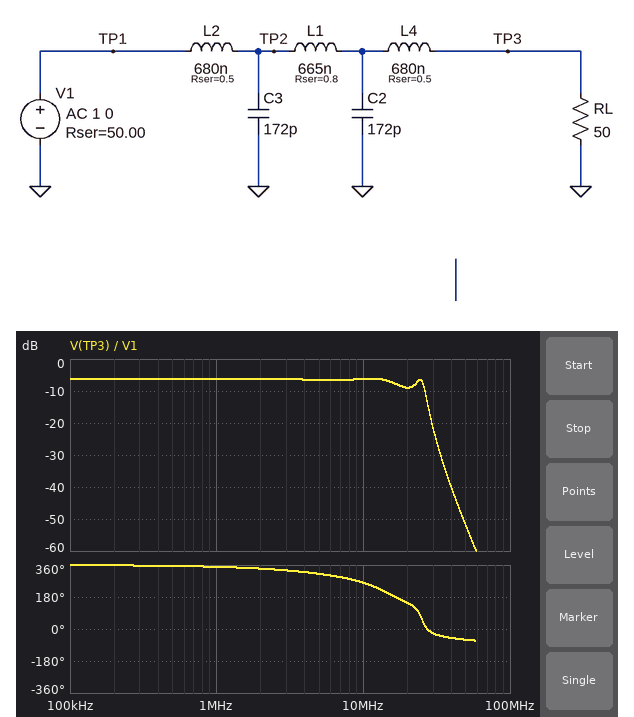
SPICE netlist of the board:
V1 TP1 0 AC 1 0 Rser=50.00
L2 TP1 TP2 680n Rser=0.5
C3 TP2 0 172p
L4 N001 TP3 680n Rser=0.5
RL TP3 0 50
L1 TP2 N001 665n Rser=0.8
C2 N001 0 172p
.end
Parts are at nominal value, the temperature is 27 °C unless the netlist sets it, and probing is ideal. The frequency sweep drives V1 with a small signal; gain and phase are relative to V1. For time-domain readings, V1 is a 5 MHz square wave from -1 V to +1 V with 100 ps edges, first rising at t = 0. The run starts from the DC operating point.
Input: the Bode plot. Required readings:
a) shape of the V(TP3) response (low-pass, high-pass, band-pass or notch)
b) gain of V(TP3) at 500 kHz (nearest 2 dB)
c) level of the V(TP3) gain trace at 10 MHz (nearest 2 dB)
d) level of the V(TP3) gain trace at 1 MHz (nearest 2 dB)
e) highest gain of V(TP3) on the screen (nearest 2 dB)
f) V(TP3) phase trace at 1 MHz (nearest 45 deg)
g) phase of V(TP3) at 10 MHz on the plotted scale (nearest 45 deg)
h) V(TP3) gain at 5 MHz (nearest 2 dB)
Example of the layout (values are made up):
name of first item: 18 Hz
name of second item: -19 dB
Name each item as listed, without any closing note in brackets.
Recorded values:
shape of the V(TP3) response: low-pass
gain of V(TP3) at 500 kHz: -6 dB
level of the V(TP3) gain trace at 10 MHz: -6 dB
level of the V(TP3) gain trace at 1 MHz: -6 dB
highest gain of V(TP3) on the screen: -6 dB
V(TP3) phase trace at 1 MHz: 360 deg
phase of V(TP3) at 10 MHz on the plotted scale: 270 deg
V(TP3) gain at 5 MHz: -6 dB
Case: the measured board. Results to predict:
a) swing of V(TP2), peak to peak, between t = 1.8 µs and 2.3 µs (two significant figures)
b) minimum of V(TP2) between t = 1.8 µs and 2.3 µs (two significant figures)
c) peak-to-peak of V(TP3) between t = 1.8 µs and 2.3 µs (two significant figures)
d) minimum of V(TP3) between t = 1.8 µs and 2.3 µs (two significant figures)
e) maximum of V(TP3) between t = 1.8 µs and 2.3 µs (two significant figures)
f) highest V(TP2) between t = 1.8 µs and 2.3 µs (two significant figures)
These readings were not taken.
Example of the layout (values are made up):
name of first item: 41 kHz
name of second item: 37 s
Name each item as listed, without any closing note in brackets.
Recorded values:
swing of V(TP2), peak to peak, between t = 1.8 µs and 2.3 µs: 1.7 V
minimum of V(TP2) between t = 1.8 µs and 2.3 µs: -850 mV
peak-to-peak of V(TP3) between t = 1.8 µs and 2.3 µs: 1.3 V
minimum of V(TP3) between t = 1.8 µs and 2.3 µs: -640 mV
maximum of V(TP3) between t = 1.8 µs and 2.3 µs: 640 mV
highest V(TP2) between t = 1.8 µs and 2.3 µs: 850 mV
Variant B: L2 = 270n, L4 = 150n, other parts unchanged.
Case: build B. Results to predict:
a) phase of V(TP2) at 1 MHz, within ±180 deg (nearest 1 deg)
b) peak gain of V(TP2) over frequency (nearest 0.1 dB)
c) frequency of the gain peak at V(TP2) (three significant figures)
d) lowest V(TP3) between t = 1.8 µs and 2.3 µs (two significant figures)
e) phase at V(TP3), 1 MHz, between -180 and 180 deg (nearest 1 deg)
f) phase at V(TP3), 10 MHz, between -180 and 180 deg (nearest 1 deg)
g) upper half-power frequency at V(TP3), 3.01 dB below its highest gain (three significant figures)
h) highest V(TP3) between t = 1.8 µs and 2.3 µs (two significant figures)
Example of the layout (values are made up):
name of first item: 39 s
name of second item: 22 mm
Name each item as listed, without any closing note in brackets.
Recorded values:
phase of V(TP2) at 1 MHz, within ±180 deg: -1 deg
peak gain of V(TP2) over frequency: -0.8 dB
frequency of the gain peak at V(TP2): 25.9 MHz
lowest V(TP3) between t = 1.8 µs and 2.3 µs: -610 mV
phase at V(TP3), 1 MHz, between -180 and 180 deg: -7 deg
phase at V(TP3), 10 MHz, between -180 and 180 deg: -71 deg
upper half-power frequency at V(TP3), 3.01 dB below its highest gain: 27.2 MHz
highest V(TP3) between t = 1.8 µs and 2.3 µs: 610 mV
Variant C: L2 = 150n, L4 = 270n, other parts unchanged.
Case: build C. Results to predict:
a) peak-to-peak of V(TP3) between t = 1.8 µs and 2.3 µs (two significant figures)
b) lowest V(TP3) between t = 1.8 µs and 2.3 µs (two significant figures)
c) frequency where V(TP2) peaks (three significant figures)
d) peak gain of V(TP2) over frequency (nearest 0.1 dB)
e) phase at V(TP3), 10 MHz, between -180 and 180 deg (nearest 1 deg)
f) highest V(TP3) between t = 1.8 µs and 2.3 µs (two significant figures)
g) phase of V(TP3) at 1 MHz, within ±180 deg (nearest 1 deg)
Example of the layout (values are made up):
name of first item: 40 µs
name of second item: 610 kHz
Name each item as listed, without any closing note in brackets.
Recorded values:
peak-to-peak of V(TP3) between t = 1.8 µs and 2.3 µs: 1.2 V
lowest V(TP3) between t = 1.8 µs and 2.3 µs: -610 mV
frequency where V(TP2) peaks: 27.7 MHz
peak gain of V(TP2) over frequency: -1.7 dB
phase at V(TP3), 10 MHz, between -180 and 180 deg: -71 deg
highest V(TP3) between t = 1.8 µs and 2.3 µs: 610 mV
phase of V(TP3) at 1 MHz, within ±180 deg: -7 deg
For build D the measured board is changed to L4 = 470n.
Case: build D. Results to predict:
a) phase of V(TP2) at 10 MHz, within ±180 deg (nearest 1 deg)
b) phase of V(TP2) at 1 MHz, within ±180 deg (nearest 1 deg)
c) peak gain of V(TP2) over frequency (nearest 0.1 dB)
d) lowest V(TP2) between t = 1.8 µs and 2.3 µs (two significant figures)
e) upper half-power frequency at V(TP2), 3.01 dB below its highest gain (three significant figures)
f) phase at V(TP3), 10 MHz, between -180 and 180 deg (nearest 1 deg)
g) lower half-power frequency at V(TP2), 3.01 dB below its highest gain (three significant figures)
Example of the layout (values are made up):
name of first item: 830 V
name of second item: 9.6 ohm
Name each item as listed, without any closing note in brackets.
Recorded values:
phase of V(TP2) at 10 MHz, within ±180 deg: -29 deg
phase of V(TP2) at 1 MHz, within ±180 deg: -2 deg
peak gain of V(TP2) over frequency: -0.8 dB
lowest V(TP2) between t = 1.8 µs and 2.3 µs: -800 mV
upper half-power frequency at V(TP2), 3.01 dB below its highest gain: 28.4 MHz
phase at V(TP3), 10 MHz, between -180 and 180 deg: -93 deg
lower half-power frequency at V(TP2), 3.01 dB below its highest gain: 23.2 MHz
